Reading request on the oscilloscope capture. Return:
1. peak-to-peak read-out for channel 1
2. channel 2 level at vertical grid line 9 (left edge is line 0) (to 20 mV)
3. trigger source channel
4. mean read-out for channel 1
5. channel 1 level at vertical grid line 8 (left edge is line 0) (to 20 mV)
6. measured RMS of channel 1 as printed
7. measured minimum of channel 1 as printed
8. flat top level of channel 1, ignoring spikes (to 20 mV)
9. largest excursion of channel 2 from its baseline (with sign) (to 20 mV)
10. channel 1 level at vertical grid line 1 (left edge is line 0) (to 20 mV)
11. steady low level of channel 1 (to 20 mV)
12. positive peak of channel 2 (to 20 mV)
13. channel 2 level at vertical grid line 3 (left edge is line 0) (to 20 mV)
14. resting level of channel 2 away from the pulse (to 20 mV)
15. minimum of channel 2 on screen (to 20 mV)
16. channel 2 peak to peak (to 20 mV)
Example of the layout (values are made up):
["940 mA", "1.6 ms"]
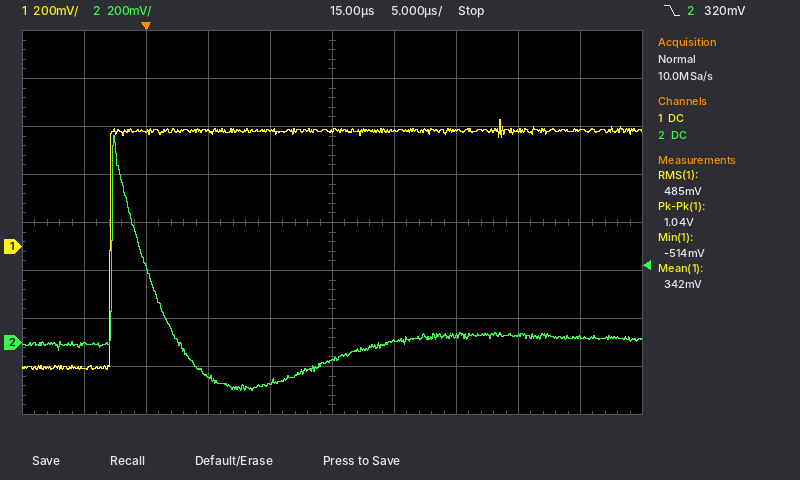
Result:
["1.04 V", "20 mV", "channel 2", "342 mV", "480 mV", "485 mV", "-514 mV", "480 mV", "+840 mV", "-500 mV", "-500 mV", "860 mV", "-140 mV", "20 mV", "-200 mV", "1.06 V"]
